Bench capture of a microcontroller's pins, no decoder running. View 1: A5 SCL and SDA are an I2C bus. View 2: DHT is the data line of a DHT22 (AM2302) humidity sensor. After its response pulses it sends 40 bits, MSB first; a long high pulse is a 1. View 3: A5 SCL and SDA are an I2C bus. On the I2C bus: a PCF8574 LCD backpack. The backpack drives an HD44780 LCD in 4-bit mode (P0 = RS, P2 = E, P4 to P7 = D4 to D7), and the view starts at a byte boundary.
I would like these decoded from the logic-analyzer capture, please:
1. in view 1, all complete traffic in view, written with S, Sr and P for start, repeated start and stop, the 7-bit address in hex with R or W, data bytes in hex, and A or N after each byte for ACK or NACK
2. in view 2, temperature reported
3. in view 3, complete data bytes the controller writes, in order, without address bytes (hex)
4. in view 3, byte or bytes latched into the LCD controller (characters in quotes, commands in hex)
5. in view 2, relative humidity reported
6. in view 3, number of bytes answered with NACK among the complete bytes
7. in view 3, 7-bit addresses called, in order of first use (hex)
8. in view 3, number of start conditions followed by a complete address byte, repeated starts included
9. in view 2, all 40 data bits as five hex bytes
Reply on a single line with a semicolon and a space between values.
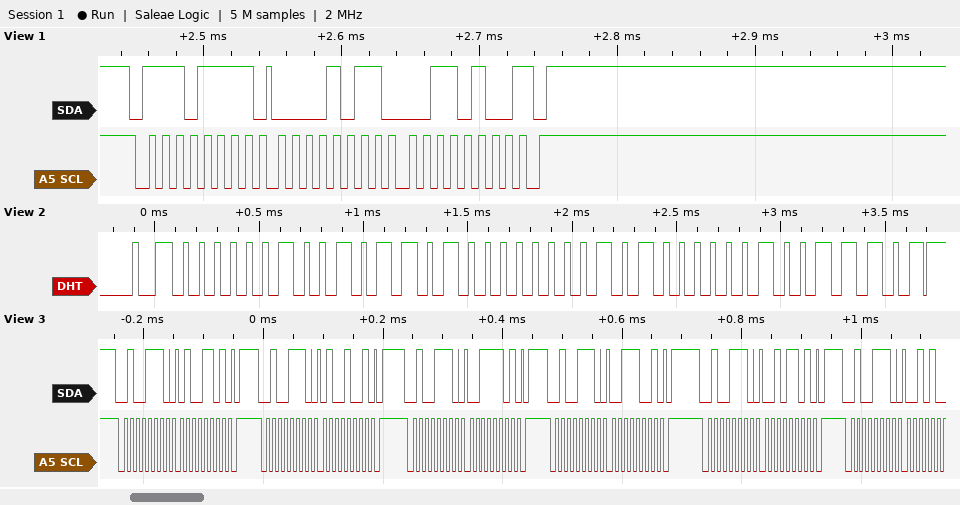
S 77R A 0B A 34 N P; 32.0 °C; 4D 49 3D 39 2D; 'C'; 60.2 %; 0; 0x27; 6; 02 5A 01 40 9D
